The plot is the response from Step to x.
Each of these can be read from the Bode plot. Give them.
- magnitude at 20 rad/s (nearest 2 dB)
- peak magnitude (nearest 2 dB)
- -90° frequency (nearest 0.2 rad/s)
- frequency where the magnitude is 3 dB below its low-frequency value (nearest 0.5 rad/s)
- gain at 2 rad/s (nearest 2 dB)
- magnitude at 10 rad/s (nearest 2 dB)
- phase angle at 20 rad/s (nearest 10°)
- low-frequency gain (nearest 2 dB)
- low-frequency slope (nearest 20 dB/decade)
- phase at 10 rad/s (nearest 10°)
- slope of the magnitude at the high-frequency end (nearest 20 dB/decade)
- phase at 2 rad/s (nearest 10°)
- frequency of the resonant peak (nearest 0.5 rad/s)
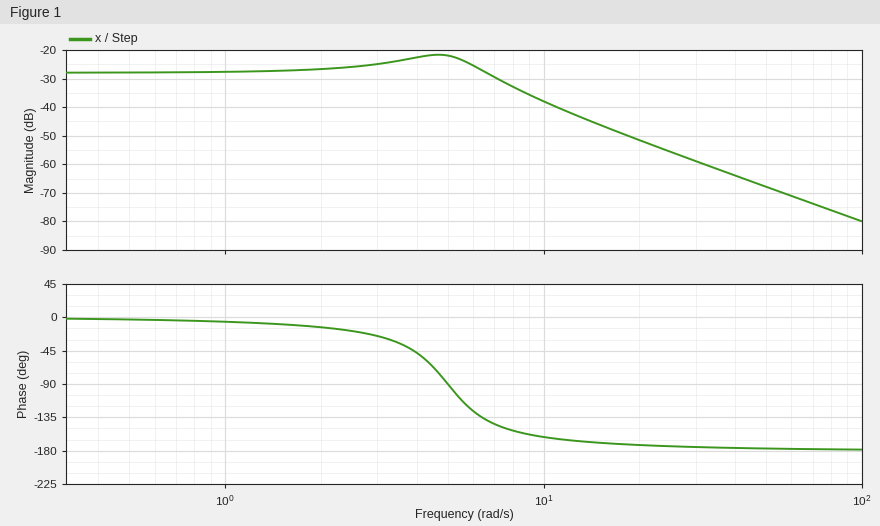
-52 dB
-22 dB
5.0 rad/s
7.5 rad/s
-26 dB
-38 dB
-170°
-28 dB
0 dB/decade
-160°
-40 dB/decade
-10°
4.5 rad/s
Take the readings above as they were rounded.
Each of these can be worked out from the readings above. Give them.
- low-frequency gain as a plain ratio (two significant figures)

0.040
